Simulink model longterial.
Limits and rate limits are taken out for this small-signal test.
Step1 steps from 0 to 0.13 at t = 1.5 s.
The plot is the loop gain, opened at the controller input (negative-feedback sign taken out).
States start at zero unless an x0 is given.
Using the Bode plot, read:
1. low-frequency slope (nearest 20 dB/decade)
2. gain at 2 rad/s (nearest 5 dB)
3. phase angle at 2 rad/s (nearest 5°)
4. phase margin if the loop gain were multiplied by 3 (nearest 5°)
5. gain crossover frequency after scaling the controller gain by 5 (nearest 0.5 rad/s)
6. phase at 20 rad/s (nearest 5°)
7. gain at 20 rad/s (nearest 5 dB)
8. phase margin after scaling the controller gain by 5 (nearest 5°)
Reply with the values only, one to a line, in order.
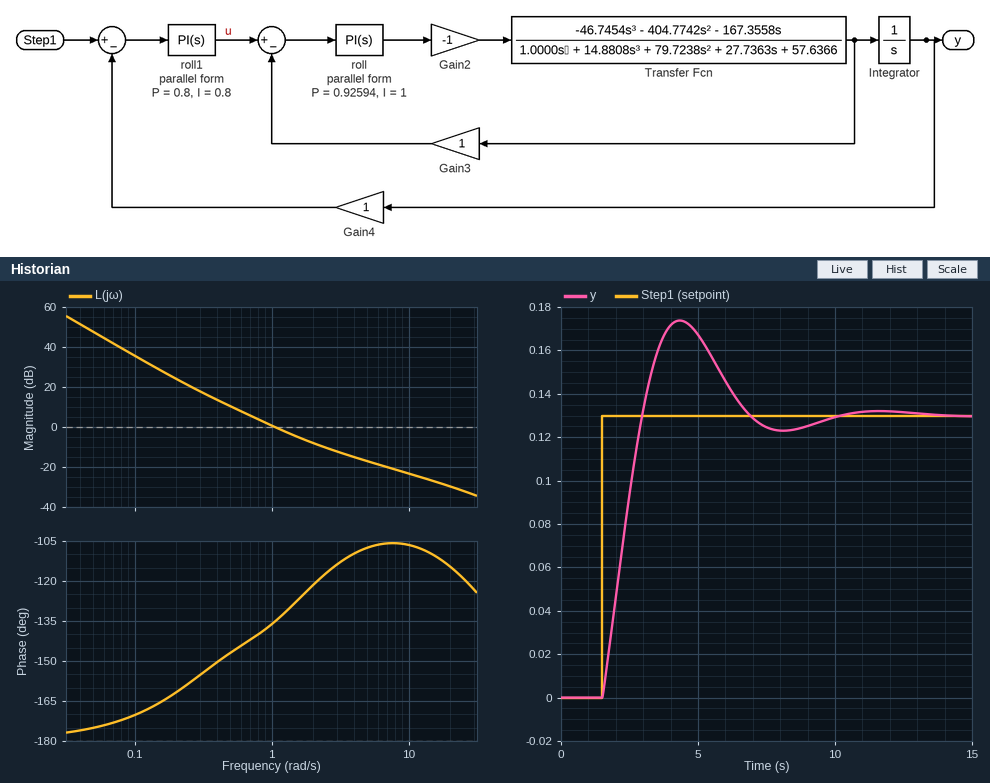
-40 dB/decade
-10 dB
-120°
60°
3.5 rad/s
-115°
-30 dB
70°
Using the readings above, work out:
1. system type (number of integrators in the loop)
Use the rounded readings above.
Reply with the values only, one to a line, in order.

2
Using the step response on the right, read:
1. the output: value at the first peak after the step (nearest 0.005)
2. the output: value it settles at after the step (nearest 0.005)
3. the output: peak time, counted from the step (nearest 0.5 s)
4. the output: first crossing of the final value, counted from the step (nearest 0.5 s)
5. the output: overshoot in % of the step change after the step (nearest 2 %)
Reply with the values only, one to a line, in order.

0.175
0.130
3.0 s
1.5 s
34 %
